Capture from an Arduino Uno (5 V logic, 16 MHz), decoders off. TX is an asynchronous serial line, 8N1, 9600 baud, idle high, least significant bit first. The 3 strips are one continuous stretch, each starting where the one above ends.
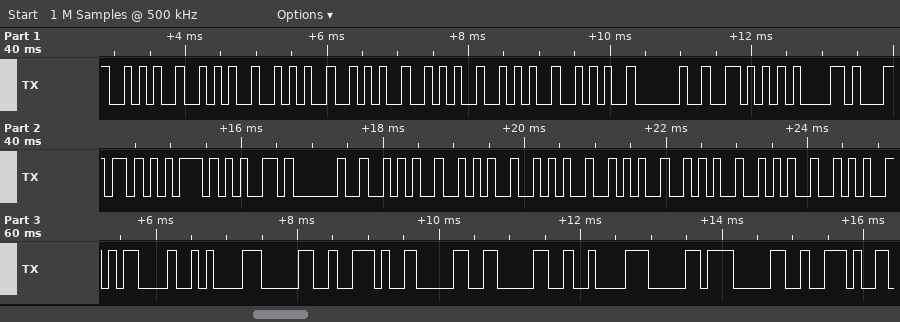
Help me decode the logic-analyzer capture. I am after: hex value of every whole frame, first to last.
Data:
2A 2A 2A 2A 2A 2A 2A 20 56 61 6C 75 65 20 2A 2A 2A 2A 2A 2A 2A 0D 0A 30 2E 30 30 C2 B0 30 2E
